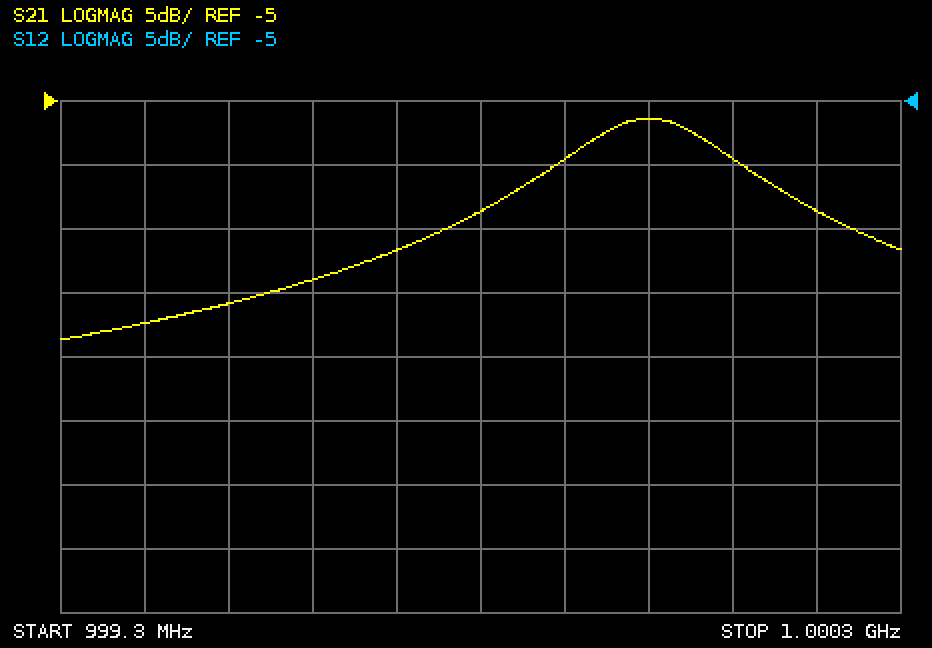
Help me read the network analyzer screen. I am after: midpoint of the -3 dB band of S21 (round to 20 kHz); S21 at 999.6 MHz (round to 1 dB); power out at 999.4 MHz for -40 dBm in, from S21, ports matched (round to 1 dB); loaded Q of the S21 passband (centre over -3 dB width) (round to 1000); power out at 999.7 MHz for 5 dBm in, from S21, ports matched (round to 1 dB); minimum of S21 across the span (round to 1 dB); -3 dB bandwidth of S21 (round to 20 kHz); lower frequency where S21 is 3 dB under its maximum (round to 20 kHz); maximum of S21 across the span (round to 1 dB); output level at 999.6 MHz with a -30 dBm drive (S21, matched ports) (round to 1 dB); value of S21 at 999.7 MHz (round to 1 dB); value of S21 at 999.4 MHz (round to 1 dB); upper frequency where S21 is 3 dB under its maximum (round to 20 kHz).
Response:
1.00000 GHz
-19 dB
-62 dBm
5000
-12 dBm
-24 dB
200 kHz
999.90 MHz
-6 dB
-49 dBm
-17 dB
-22 dB
1.00010 GHz
